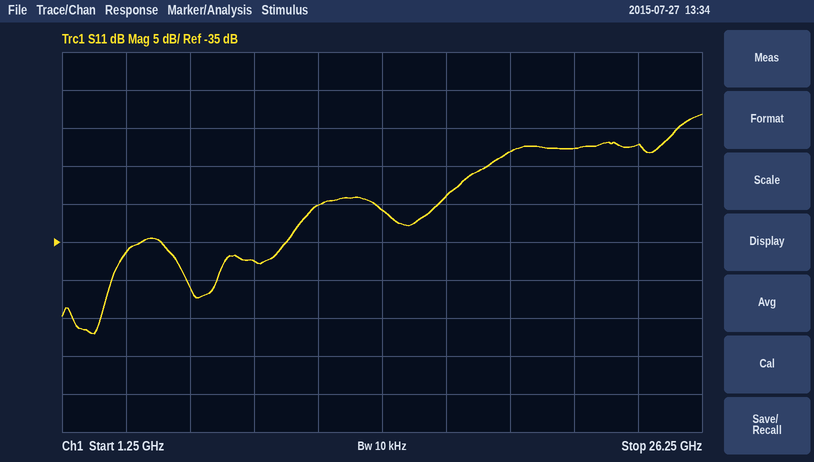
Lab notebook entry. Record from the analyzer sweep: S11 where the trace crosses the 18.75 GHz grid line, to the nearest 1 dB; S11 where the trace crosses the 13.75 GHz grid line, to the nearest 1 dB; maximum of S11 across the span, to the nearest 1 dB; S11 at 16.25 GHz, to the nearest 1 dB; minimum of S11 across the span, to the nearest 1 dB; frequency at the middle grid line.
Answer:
-23 dB
-31 dB
-18 dB
-29 dB
-47 dB
13.75 GHz
